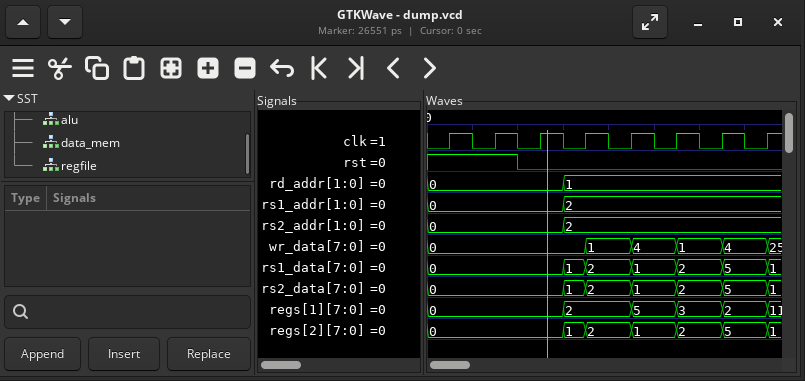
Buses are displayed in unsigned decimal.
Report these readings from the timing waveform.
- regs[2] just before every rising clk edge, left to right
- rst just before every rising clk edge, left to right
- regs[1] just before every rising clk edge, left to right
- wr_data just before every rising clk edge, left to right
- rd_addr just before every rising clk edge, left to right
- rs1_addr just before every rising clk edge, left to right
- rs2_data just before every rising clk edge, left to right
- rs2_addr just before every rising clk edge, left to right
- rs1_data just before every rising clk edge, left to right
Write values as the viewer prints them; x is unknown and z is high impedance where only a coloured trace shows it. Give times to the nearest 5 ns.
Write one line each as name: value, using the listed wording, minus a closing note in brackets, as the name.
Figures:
regs[2] just before every rising clk edge, left to right: 0, 0, 0, 1, 2, 1, 2, 5
rst just before every rising clk edge, left to right: 1 1 0 0 0 0 0 0
regs[1] just before every rising clk edge, left to right: 0, 0, 0, 2, 2, 5, 3, 2
wr_data just before every rising clk edge, left to right: 0, 0, 0, 0, 1, 4, 1, 4
rd_addr just before every rising clk edge, left to right: 0, 0, 0, 1, 1, 1, 1, 1
rs1_addr just before every rising clk edge, left to right: 0, 0, 0, 2, 2, 2, 2, 2
rs2_data just before every rising clk edge, left to right: 0, 0, 0, 1, 2, 1, 2, 5
rs2_addr just before every rising clk edge, left to right: 0, 0, 0, 2, 2, 2, 2, 2
rs1_data just before every rising clk edge, left to right: 0, 0, 0, 1, 2, 1, 2, 5
